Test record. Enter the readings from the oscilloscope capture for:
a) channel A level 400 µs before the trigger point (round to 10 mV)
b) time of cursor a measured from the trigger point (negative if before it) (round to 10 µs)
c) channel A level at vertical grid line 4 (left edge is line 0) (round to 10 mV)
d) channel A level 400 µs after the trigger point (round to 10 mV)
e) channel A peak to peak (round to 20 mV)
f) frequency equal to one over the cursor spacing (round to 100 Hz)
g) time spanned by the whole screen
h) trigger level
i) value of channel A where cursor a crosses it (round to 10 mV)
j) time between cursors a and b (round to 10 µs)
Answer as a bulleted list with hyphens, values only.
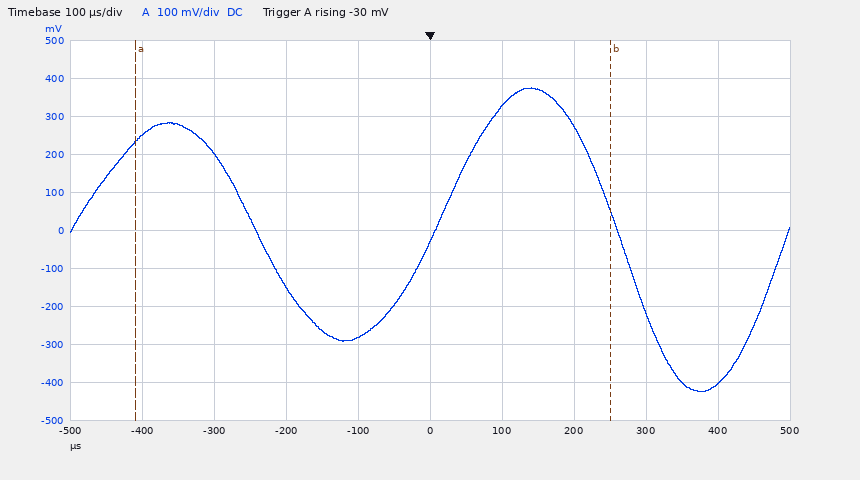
- 250 mV
- -410 µs
- -280 mV
- -400 mV
- 800 mV
- 1.5 kHz
- 1 ms
- -30 mV
- 230 mV
- 660 µs
